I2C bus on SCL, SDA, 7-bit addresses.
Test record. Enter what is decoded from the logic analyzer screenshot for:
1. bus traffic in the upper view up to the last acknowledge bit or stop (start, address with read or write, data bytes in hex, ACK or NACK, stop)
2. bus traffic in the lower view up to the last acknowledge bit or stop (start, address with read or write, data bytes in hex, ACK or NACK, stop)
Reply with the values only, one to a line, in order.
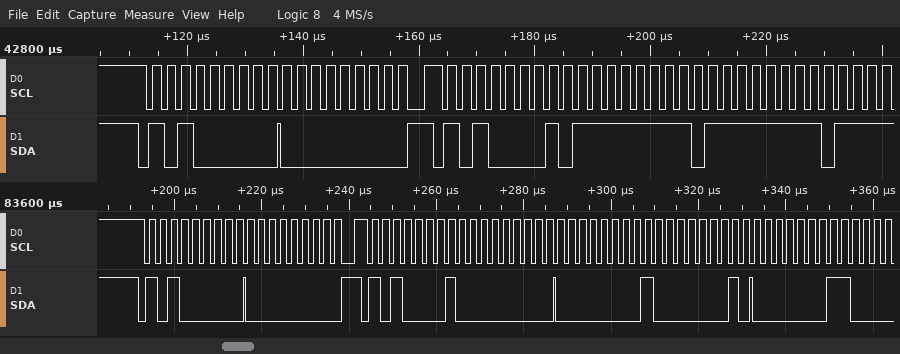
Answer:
start, address 50 write ACK, 00 ACK, repeated start, address 50 read ACK, FF ACK, FF ACK
start, address 50 write ACK, 00 ACK, repeated start, address 50 read ACK, 00 ACK, 01 ACK, 02 ACK, 03 ACK
